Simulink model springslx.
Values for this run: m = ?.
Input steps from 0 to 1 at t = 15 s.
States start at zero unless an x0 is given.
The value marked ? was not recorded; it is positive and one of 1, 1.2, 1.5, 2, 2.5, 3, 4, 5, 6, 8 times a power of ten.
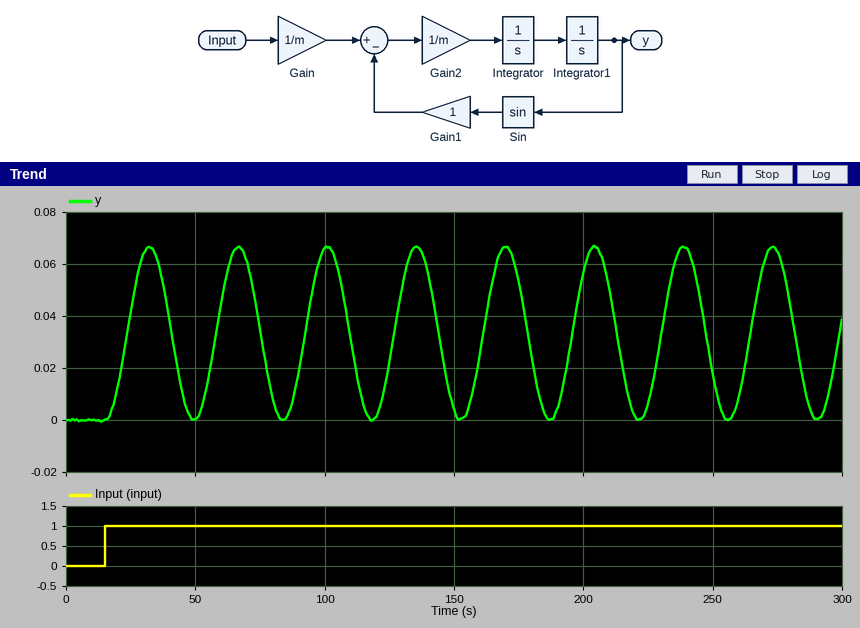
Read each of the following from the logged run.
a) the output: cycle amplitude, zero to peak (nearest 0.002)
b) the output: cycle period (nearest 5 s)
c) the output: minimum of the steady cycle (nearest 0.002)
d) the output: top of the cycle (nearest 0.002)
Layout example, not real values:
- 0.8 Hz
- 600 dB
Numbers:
- 0.034
- 35 s
- 0.000
- 0.066
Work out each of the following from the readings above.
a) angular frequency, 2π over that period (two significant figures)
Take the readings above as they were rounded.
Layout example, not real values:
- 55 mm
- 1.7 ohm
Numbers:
- 0.18 rad/s
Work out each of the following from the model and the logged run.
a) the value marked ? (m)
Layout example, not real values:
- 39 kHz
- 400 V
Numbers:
- 30
